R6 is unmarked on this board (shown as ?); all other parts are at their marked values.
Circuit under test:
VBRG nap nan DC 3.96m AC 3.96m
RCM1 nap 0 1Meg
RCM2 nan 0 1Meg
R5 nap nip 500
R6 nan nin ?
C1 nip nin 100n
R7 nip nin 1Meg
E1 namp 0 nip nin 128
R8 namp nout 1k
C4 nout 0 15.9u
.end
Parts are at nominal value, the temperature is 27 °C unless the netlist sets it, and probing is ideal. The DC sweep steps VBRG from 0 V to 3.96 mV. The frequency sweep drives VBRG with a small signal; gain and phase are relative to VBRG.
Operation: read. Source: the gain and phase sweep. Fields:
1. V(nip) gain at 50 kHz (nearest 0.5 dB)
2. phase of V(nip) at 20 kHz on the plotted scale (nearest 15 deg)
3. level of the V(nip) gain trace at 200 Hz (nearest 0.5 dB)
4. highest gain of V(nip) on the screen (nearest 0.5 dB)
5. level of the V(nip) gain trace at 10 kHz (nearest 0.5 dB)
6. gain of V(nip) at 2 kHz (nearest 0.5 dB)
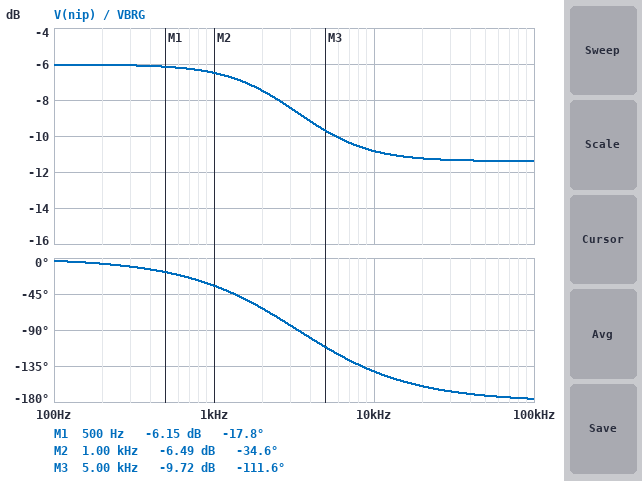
-11.5 dB
-165 deg
-6.0 dB
-6.0 dB
-11.0 dB
-7.5 dB
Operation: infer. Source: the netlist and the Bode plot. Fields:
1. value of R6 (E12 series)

150 Ω
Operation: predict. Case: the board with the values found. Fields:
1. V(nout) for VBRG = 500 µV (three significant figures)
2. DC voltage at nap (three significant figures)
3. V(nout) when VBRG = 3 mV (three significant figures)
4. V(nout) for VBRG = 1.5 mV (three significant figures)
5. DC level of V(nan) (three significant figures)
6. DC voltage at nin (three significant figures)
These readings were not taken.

64.0 mV
1.98 mV
384 mV
192 mV
-1.98 mV
-1.98 mV
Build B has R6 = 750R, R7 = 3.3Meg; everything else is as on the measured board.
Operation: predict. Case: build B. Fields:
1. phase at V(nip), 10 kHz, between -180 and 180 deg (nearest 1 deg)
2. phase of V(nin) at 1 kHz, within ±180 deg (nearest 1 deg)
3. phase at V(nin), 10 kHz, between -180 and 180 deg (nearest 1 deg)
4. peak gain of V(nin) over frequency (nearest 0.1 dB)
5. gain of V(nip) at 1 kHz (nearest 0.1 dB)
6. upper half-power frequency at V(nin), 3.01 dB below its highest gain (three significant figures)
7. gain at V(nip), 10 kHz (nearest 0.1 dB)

-25 deg
133 deg
40 deg
-6.0 dB
-8.0 dB
1.33 kHz
-18.6 dB
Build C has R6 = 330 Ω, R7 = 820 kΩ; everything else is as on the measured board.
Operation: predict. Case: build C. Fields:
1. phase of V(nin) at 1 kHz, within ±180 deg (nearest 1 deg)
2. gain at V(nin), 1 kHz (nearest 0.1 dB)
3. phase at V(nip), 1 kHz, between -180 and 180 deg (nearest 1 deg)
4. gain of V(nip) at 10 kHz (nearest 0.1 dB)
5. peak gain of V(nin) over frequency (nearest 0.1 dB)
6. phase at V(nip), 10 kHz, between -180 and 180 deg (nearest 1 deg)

159 deg
-7.0 dB
-34 deg
-17.2 dB
-6.0 dB
-126 deg
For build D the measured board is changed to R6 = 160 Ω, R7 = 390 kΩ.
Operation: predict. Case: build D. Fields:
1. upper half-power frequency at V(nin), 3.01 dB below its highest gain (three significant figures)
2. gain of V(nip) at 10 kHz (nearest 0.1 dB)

3.53 kHz
-11.2 dB
